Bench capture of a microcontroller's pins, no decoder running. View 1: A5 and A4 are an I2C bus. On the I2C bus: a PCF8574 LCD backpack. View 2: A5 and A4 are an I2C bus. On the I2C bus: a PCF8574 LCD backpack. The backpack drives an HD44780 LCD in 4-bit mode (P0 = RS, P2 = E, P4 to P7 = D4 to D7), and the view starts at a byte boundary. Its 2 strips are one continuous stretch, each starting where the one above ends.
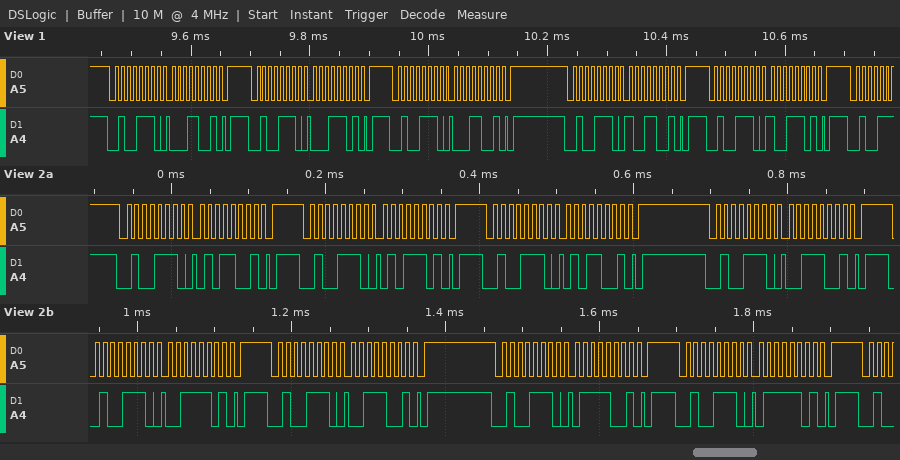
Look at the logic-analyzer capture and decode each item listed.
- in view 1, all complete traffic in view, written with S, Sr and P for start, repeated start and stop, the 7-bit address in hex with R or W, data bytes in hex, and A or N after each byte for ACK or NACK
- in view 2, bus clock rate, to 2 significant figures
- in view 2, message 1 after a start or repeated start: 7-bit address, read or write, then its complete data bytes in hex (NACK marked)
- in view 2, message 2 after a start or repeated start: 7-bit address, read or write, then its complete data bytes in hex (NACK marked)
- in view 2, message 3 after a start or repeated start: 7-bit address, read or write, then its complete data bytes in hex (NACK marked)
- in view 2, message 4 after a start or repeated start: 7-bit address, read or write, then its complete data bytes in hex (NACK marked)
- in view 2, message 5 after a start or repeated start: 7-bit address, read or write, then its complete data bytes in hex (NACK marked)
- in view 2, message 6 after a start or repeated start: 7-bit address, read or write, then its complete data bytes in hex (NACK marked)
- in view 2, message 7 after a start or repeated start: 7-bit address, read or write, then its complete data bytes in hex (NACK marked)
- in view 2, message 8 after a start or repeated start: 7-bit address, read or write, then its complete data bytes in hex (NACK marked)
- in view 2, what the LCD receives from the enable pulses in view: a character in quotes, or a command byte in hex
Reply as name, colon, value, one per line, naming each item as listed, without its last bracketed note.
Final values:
in view 1, all complete traffic in view, written with S, Sr and P for start, repeated start and stop, the 7-bit address in hex with R or W, data bytes in hex, and A or N after each byte for ACK or NACK: S 27W A 19 A P S 27W A 1D A P S 27W A 19 A P S 27W A 99 A P S 27W A 9D A P
in view 2, bus clock rate, to 2 significant figures: 100 kHz
in view 2, message 1 after a start or repeated start: 7-bit address, read or write, then its complete data bytes in hex: 0x27 write: 59
in view 2, message 2 after a start or repeated start: 7-bit address, read or write, then its complete data bytes in hex: 0x27 write: 5D
in view 2, message 3 after a start or repeated start: 7-bit address, read or write, then its complete data bytes in hex: 0x27 write: 59
in view 2, message 4 after a start or repeated start: 7-bit address, read or write, then its complete data bytes in hex: 0x27 write: 39
in view 2, message 5 after a start or repeated start: 7-bit address, read or write, then its complete data bytes in hex: 0x27 write: 3D
in view 2, message 6 after a start or repeated start: 7-bit address, read or write, then its complete data bytes in hex: 0x27 write: 39
in view 2, message 7 after a start or repeated start: 7-bit address, read or write, then its complete data bytes in hex: 0x27 write: 79
in view 2, message 8 after a start or repeated start: 7-bit address, read or write, then its complete data bytes in hex: 0x27 write: 7D
in view 2, what the LCD receives from the enable pulses in view: a character in quotes, or a command byte in hex: 'S'
